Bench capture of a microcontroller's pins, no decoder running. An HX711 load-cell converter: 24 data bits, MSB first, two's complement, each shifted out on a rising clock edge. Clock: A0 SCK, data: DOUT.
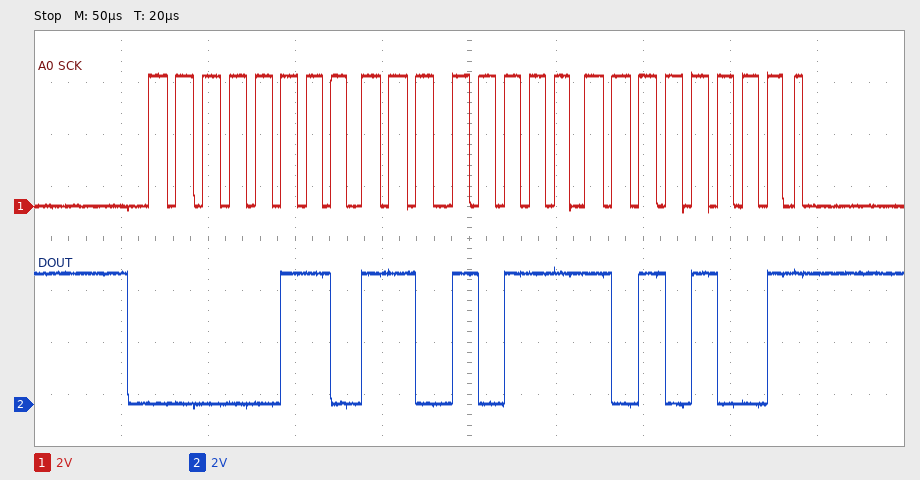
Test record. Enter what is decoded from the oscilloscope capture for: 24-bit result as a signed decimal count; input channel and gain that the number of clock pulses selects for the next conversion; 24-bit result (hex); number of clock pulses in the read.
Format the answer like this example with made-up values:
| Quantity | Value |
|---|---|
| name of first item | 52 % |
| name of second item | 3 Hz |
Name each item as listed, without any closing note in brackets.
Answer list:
| Quantity | Value |
|---|---|
| 24-bit result as a signed decimal count | 448425 |
| input channel and gain that the number of clock pulses selects for the next conversion | channel A, gain 128 |
| 24-bit result | 0x06D7A9 |
| number of clock pulses in the read | 25 |
